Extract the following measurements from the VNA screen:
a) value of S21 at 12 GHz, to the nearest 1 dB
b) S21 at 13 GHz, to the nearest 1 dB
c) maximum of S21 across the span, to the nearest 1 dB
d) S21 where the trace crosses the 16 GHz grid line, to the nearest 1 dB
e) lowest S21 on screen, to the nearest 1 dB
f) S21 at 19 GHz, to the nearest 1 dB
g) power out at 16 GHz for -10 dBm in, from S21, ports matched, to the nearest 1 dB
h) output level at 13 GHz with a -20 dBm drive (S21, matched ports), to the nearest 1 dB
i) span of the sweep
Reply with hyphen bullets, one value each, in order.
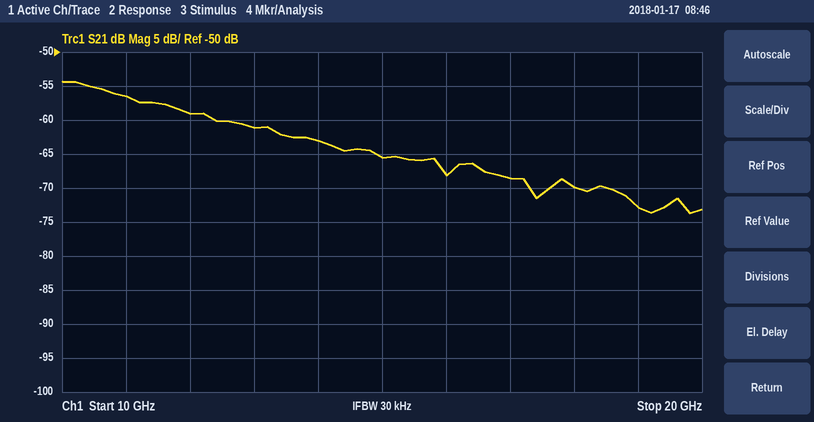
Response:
- -59 dB
- -61 dB
- -54 dB
- -68 dB
- -74 dB
- -73 dB
- -78 dBm
- -81 dBm
- 10 GHz
